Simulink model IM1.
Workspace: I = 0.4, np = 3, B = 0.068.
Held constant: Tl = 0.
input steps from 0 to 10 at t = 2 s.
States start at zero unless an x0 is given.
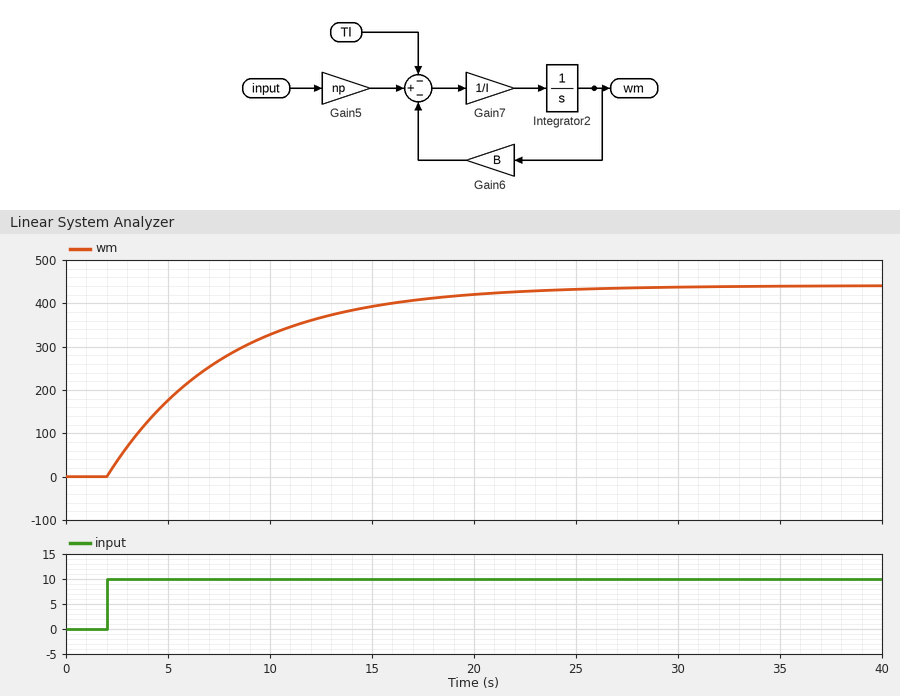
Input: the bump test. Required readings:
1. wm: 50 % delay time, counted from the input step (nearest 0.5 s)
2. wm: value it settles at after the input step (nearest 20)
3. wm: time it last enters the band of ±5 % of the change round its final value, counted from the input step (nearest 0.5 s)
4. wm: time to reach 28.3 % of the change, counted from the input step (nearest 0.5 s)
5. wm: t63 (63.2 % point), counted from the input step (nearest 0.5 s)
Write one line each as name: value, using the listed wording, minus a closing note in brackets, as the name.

wm: 50 % delay time, counted from the input step: 4.0 s
wm: value it settles at after the input step: 440
wm: time it last enters the band of ±5 % of the change round its final value, counted from the input step: 17.5 s
wm: time to reach 28.3 % of the change, counted from the input step: 2.0 s
wm: t63 (63.2 % point), counted from the input step: 6.0 s
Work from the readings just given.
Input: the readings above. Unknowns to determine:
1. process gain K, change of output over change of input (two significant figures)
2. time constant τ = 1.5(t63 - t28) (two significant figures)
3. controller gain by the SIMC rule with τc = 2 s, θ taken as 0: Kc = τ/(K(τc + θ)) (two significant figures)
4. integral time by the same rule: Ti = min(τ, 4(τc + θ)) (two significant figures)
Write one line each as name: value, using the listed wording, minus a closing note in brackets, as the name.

process gain K, change of output over change of input: 44
time constant τ = 1.5(t63 - t28): 6.0 s
controller gain by the SIMC rule with τc = 2 s, θ taken as 0: Kc = τ/(K(τc + θ)): 0.068
integral time by the same rule: Ti = min(τ, 4(τc + θ)): 6.0 s
